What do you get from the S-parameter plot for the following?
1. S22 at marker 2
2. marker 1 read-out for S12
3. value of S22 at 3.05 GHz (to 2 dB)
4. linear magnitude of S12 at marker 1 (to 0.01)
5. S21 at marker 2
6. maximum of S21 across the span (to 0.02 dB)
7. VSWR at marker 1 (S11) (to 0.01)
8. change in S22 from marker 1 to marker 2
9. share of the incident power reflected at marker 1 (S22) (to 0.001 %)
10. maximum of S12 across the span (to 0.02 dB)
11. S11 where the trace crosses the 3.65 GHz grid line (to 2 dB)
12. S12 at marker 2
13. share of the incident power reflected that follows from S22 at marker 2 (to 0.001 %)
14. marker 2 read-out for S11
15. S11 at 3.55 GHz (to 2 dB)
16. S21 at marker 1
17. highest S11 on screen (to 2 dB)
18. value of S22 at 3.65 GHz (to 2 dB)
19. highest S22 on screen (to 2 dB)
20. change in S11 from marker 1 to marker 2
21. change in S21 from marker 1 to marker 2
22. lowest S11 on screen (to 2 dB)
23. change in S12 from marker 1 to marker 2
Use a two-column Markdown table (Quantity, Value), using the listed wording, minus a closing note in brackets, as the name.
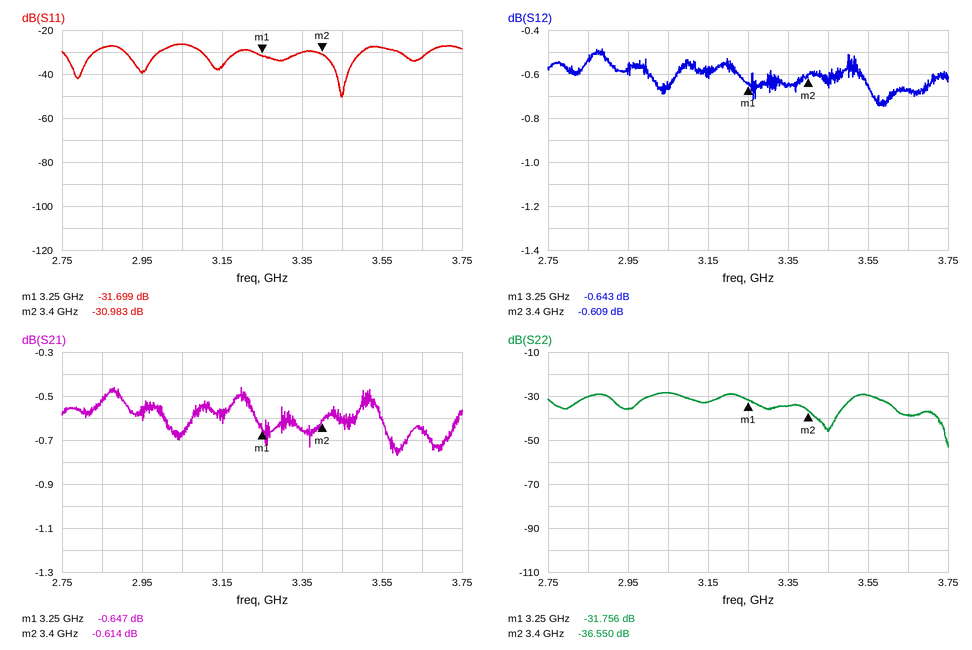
| Quantity | Value |
|---|---|
| S22 at marker 2 | -36.550 dB |
| marker 1 read-out for S12 | -0.643 dB |
| value of S22 at 3.05 GHz | -28 dB |
| linear magnitude of S12 at marker 1 | 0.93 |
| S21 at marker 2 | -0.614 dB |
| maximum of S21 across the span | -0.46 dB |
| VSWR at marker 1 (S11) | 1.05 |
| change in S22 from marker 1 to marker 2 | -4.794 dB |
| share of the incident power reflected at marker 1 (S22) | 0.067 % |
| maximum of S12 across the span | -0.48 dB |
| S11 where the trace crosses the 3.65 GHz grid line | -32 dB |
| S12 at marker 2 | -0.609 dB |
| share of the incident power reflected that follows from S22 at marker 2 | 0.022 % |
| marker 2 read-out for S11 | -30.983 dB |
| S11 at 3.55 GHz | -28 dB |
| S21 at marker 1 | -0.647 dB |
| highest S11 on screen | -26 dB |
| value of S22 at 3.65 GHz | -38 dB |
| highest S22 on screen | -28 dB |
| change in S11 from marker 1 to marker 2 | 0.716 dB |
| change in S21 from marker 1 to marker 2 | 0.033 dB |
| lowest S11 on screen | -50 dB |
| change in S12 from marker 1 to marker 2 | 0.034 dB |
